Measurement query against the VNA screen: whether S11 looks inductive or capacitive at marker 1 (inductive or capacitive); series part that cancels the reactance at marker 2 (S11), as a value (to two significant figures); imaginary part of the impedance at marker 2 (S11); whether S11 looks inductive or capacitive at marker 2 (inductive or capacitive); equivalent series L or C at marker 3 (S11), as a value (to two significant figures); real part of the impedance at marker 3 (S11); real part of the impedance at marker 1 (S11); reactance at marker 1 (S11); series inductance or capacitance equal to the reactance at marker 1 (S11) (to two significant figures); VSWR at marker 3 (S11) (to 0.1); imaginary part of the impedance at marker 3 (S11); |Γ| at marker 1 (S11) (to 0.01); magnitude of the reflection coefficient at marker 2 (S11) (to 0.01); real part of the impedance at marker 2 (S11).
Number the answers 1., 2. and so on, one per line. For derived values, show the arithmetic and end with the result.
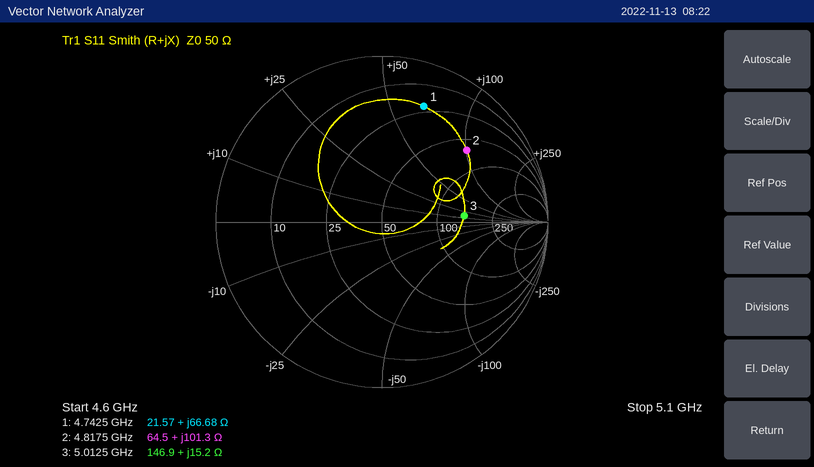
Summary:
1. inductive
2. C = 1/(2π × 4.8175 GHz × 101.3 Ω) ≈ 326 fF, so 330 fF to two significant figures
3. +101.3 Ω
4. inductive
5. L = 15.2 Ω/(2π × 5.0125 GHz) ≈ 483 pH, so 480 pH to two significant figures
6. 146.9 Ω
7. 21.57 Ω
8. +66.68 Ω
9. L = 66.68 Ω/(2π × 4.7425 GHz) ≈ 2.2 nH
10. 3.0
11. +15.2 Ω
12. 0.74
13. 0.67
14. 64.5 Ω
